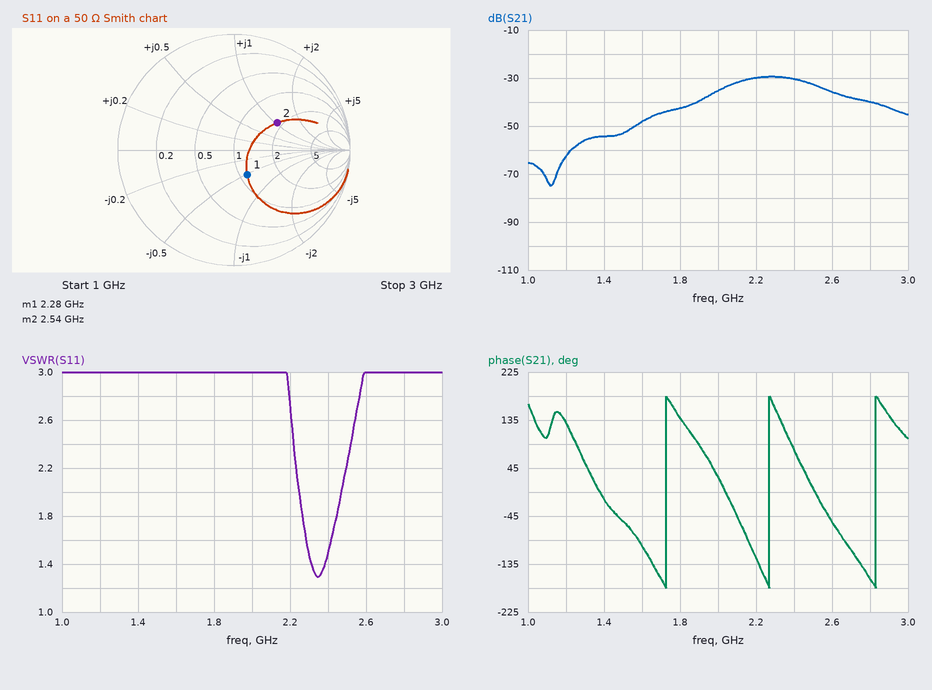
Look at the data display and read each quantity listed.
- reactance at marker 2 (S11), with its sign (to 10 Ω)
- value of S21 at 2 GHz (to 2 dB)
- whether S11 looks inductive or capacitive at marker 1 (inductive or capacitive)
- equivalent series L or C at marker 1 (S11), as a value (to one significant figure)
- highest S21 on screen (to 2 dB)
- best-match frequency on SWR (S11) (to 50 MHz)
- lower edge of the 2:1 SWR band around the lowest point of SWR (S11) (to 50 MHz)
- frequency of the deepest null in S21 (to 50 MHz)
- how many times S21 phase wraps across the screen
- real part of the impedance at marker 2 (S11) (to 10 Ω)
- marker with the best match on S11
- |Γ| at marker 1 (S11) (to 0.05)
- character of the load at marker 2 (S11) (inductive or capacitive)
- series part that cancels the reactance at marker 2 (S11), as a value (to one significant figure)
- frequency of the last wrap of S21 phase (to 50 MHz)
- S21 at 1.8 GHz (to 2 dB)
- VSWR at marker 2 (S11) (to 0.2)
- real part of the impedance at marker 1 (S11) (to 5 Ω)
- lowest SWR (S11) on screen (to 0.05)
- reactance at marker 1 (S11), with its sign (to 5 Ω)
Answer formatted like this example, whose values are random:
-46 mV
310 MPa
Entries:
+50 Ω
-36 dB
capacitive
3 pF
-30 dB
2.35 GHz
2.25 GHz
1.10 GHz
3
90 Ω
marker 1
0.25
inductive
1 pF
2.85 GHz
-42 dB
2.6
55 Ω
1.30
-25 Ω
